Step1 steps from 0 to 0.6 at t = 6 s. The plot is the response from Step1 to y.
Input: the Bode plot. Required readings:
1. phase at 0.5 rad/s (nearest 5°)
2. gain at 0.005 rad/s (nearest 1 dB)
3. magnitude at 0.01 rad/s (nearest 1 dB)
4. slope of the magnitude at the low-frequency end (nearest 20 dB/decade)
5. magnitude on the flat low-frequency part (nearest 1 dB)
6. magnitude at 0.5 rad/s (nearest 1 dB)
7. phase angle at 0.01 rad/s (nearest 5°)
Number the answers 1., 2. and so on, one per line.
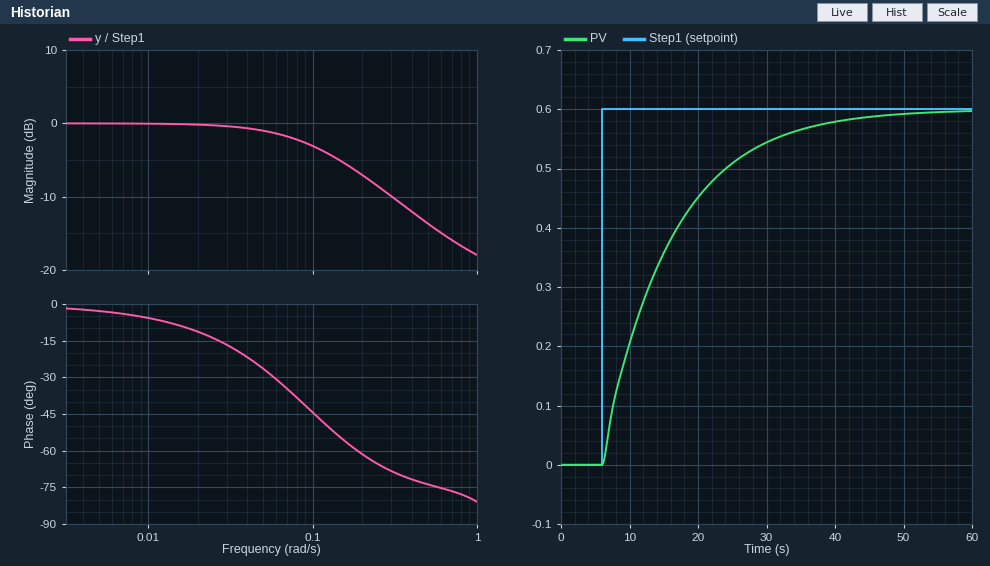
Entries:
1. -75°
2. 0 dB
3. 0 dB
4. 0 dB/decade
5. 0 dB
6. -14 dB
7. -5°
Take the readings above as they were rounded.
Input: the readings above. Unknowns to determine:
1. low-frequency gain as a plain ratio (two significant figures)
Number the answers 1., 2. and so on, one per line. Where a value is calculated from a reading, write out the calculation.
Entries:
1. 10^(0 / 20) = 1.0
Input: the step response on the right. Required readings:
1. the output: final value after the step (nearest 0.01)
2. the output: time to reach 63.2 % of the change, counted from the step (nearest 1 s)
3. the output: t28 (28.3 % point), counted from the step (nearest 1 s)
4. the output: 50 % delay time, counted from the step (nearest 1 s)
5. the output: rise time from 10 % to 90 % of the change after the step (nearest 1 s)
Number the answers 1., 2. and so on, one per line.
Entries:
1. 0.60
2. 10 s
3. 3 s
4. 7 s
5. 22 s
